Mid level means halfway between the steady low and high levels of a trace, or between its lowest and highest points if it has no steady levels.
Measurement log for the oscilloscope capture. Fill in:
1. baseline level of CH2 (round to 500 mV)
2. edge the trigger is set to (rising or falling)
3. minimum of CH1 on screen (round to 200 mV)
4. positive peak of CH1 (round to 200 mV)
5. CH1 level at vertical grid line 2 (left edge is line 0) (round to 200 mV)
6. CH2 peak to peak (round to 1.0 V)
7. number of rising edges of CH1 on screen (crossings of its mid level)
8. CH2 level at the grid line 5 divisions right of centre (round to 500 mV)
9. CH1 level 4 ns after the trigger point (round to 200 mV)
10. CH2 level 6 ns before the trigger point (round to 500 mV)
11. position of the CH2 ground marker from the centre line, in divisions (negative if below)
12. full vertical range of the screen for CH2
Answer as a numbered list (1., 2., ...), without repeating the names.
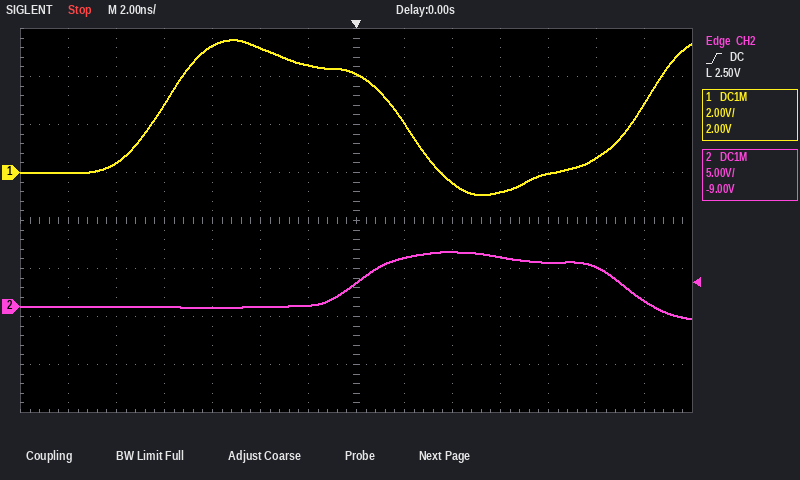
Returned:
1. 0.0 V
2. rising
3. -1.0 V
4. 5.6 V
5. 400 mV
6. 7.0 V
7. 2
8. 4.0 V
9. -400 mV
10. 0.0 V
11. -1.8 div
12. 40 V
